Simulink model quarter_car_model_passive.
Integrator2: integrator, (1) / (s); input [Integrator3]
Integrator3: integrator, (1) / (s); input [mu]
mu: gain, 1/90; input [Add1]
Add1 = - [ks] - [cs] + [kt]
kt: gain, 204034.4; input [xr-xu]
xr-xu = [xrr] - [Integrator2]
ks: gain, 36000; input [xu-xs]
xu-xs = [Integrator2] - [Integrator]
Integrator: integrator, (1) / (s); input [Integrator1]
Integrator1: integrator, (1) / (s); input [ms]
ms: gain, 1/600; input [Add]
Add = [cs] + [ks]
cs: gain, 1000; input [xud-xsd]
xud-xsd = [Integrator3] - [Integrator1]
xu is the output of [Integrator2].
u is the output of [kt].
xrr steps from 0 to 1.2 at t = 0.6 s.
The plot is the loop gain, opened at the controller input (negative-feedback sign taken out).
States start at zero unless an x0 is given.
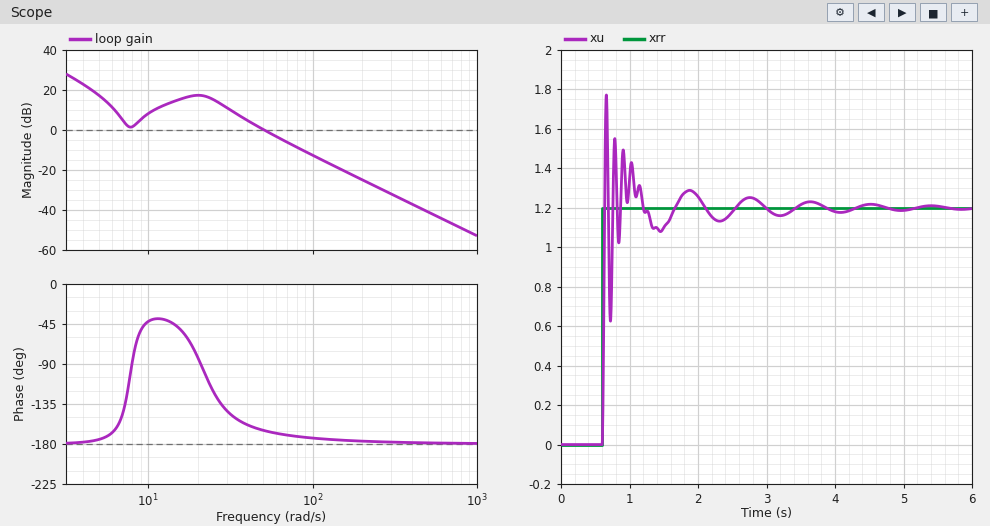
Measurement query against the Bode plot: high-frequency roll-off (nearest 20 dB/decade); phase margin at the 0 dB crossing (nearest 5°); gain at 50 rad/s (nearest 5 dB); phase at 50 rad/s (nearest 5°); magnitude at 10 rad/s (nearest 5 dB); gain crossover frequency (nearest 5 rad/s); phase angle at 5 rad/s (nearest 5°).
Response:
-40 dB/decade
15°
0 dB
-165°
10 dB
50 rad/s
-175°
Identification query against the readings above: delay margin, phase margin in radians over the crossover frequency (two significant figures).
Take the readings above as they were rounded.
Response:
0.0052 s
